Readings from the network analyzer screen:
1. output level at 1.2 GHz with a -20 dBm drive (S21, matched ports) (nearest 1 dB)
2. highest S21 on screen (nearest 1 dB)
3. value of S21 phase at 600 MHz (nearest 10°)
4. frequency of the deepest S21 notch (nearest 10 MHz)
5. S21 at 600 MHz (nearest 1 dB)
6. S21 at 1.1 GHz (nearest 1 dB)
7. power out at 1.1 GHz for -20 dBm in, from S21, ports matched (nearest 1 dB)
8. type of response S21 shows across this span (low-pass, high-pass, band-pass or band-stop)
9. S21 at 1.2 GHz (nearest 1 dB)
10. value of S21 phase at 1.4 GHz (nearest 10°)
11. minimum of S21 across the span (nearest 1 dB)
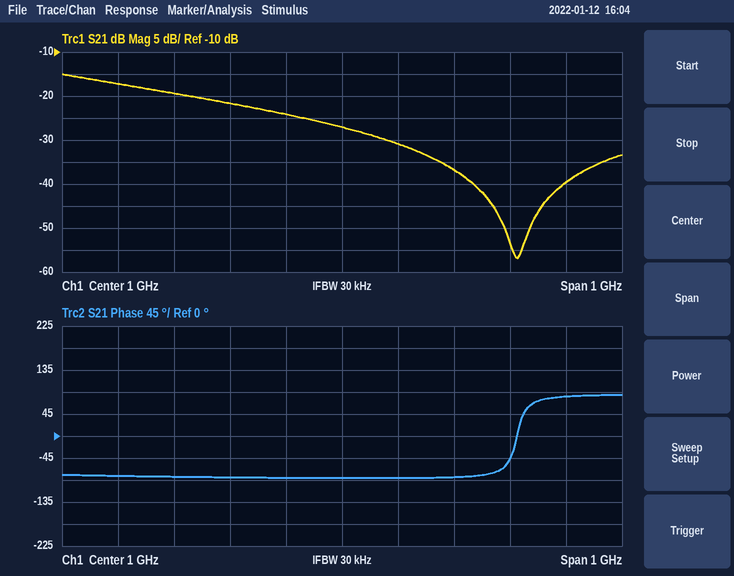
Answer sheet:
-57 dBm
-15 dB
-80°
1.31 GHz
-17 dB
-31 dB
-51 dBm
low-pass
-37 dB
80°
-57 dB
